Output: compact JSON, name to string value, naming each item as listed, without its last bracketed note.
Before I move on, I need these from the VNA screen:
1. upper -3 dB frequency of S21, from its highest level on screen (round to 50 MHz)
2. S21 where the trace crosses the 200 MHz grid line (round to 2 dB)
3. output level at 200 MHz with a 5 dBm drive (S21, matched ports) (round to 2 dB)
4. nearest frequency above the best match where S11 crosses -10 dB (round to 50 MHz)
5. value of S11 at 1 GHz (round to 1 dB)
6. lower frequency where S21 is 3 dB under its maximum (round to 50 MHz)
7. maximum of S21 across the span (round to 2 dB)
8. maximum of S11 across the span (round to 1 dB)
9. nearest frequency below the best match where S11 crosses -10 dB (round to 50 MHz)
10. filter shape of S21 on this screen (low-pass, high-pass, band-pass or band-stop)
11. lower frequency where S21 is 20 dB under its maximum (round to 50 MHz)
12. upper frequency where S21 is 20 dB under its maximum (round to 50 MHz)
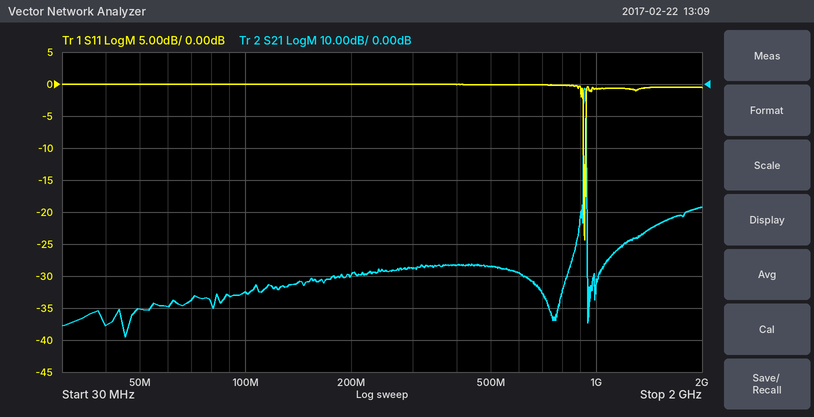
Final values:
{"upper -3 dB frequency of S21, from its highest level on screen": "950 MHz", "S21 where the trace crosses the 200 MHz grid line": "-60 dB", "output level at 200 MHz with a 5 dBm drive (S21, matched ports)": "-54 dBm", "nearest frequency above the best match where S11 crosses -10 dB": "950 MHz", "value of S11 at 1 GHz": "-1 dB", "lower frequency where S21 is 3 dB under its maximum": "900 MHz", "maximum of S21 across the span": "-2 dB", "maximum of S11 across the span": "0 dB", "nearest frequency below the best match where S11 crosses -10 dB": "900 MHz", "filter shape of S21 on this screen": "band-pass", "lower frequency where S21 is 20 dB under its maximum": "900 MHz", "upper frequency where S21 is 20 dB under its maximum": "950 MHz"}
